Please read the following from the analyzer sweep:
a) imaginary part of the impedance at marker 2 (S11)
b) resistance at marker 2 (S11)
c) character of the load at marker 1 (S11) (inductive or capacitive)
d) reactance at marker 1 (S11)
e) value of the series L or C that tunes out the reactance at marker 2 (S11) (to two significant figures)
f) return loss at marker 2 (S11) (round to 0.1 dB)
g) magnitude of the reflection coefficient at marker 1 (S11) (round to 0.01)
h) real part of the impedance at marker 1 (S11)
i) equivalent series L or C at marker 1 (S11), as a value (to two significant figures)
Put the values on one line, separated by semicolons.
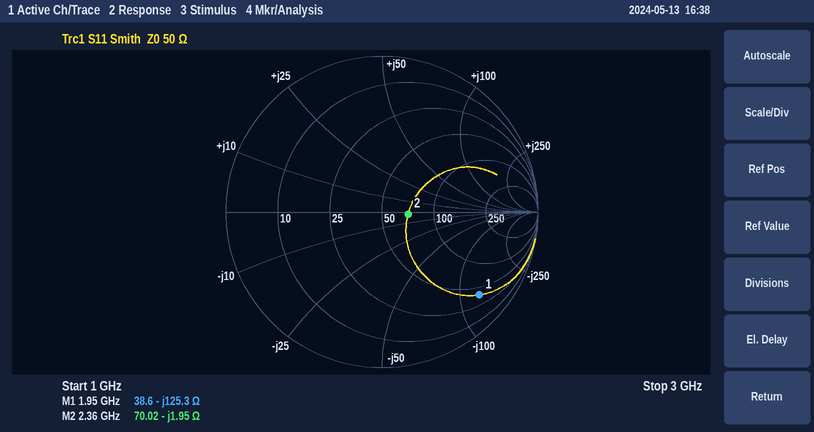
-1.95 Ω; 70.02 Ω; capacitive; -125.3 Ω; 130 pH; 15.5 dB; 0.82; 38.6 Ω; 650 fF
